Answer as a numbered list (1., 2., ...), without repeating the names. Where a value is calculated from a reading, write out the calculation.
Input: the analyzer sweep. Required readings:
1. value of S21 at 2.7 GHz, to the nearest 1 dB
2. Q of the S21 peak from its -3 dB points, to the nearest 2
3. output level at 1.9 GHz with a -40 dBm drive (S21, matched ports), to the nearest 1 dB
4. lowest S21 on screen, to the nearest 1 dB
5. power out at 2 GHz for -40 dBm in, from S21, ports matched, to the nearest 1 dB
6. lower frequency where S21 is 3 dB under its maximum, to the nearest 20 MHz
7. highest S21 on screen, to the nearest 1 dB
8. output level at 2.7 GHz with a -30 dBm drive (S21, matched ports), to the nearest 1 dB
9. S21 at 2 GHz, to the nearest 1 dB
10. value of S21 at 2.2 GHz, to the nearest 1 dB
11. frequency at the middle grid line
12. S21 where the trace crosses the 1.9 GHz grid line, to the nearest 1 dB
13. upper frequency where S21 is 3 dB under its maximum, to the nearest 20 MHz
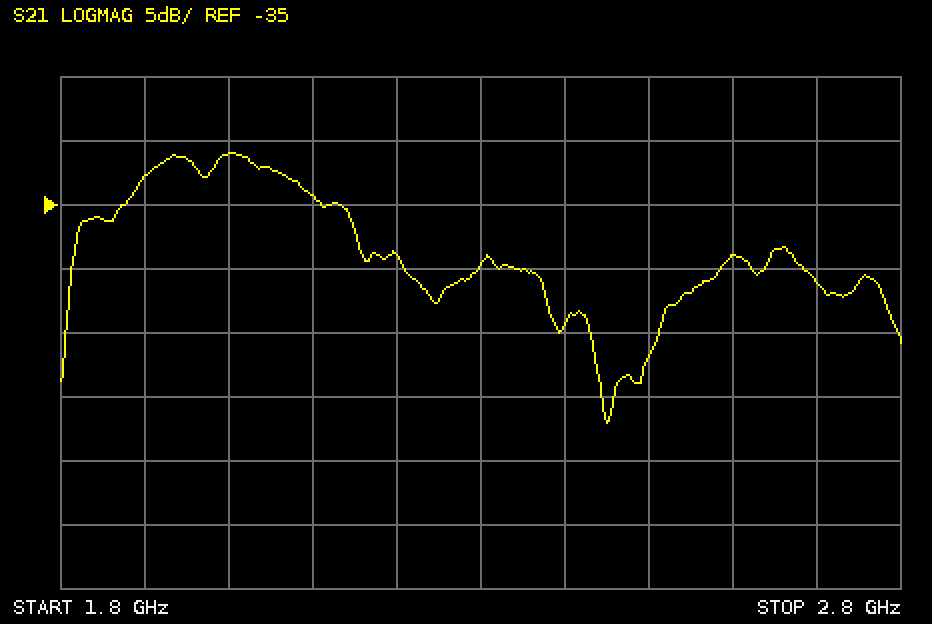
1. -41 dB
2. 1.99 GHz / 220 MHz ≈ 9.05, so 10 to the nearest 2
3. -40 dBm + (-33 dB) = -73 dBm
4. -52 dB
5. -40 dBm + (-31 dB) = -71 dBm
6. 1.88 GHz
7. -31 dB
8. -30 dBm + (-41 dB) = -71 dBm
9. -31 dB
10. -39 dB
11. 2.3 GHz
12. -33 dB
13. 2.10 GHz
